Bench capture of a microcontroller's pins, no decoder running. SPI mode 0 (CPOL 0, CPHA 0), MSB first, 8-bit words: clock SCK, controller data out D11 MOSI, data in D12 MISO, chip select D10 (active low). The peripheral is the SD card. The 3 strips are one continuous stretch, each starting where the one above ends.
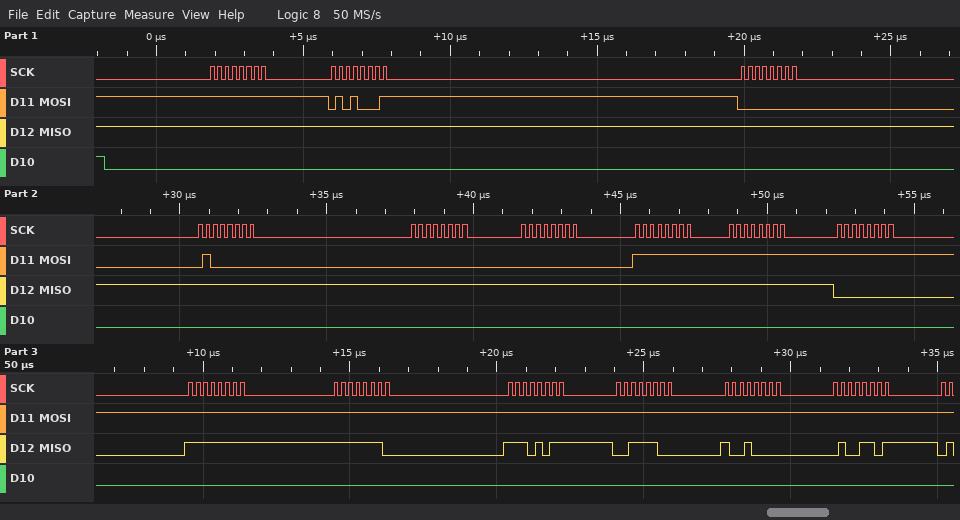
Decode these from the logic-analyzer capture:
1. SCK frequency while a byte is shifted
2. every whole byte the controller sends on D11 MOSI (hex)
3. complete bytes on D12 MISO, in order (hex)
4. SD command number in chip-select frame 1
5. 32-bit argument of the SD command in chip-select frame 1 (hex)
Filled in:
4 MHz
0xFF 0x51 0x00 0x40 0x00 0x00 0xFF 0xFF 0xFF 0xFF 0xFF 0xFF 0xFF 0xFF 0xFF
0xFF 0xFF 0xFF 0xFF 0xFF 0xFF 0xFF 0xFF 0x00 0xFF 0xFE 0xEB 0x3C 0x90 0x4D
CMD17
0x00400000
